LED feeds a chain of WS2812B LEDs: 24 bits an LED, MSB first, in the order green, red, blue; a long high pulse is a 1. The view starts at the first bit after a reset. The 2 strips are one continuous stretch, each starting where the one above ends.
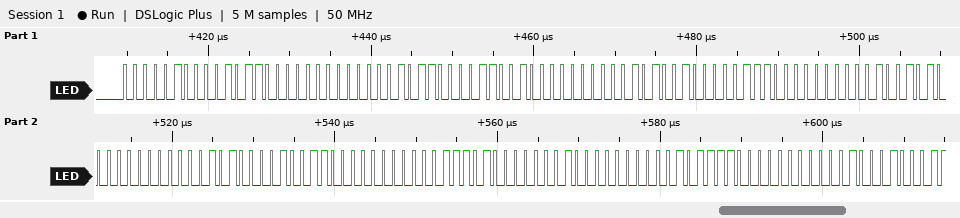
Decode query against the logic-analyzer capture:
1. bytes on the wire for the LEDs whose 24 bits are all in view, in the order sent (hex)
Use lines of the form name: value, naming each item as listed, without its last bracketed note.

bytes on the wire for the LEDs whose 24 bits are all in view, in the order sent: 04 2C 00 16 19 00 29 07 00 25 00 0A 13 00 1D 01 00 2F
